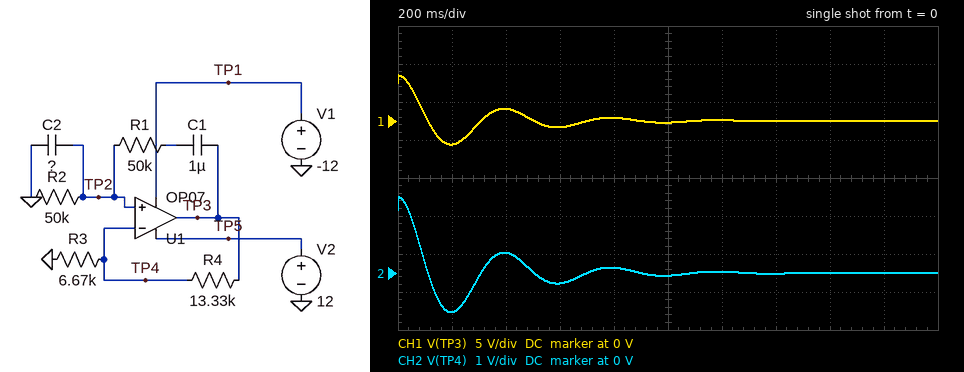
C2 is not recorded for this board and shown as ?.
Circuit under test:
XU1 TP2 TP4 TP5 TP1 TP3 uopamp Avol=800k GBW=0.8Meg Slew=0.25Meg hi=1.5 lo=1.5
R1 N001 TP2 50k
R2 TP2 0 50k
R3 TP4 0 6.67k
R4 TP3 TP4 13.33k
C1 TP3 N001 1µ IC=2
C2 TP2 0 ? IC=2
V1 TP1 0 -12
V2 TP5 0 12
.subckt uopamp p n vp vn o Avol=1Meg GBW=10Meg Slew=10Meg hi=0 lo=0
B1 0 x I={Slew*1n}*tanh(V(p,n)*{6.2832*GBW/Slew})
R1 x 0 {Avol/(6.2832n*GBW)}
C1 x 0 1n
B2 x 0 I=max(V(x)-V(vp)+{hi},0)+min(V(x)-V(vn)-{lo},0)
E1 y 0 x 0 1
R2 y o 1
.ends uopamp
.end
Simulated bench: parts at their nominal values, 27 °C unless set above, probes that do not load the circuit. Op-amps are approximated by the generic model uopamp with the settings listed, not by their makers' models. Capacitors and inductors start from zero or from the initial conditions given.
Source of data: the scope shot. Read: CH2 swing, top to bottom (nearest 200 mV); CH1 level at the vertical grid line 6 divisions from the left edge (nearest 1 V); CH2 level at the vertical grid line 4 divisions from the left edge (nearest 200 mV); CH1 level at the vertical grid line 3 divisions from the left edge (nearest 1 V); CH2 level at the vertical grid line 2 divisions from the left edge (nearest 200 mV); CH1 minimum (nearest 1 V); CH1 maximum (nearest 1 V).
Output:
3.0 V
0 V
200 mV
-1 V
600 mV
-3 V
6 V
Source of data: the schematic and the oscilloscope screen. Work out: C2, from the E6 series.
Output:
1.5 µF
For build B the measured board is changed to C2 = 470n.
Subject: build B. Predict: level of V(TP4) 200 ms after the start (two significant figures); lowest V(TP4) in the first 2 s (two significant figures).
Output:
3.5 V
-3.5 V
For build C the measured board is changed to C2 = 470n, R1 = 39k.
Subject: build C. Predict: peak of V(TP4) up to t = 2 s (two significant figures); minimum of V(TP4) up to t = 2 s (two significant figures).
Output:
3.5 V
-3.5 V
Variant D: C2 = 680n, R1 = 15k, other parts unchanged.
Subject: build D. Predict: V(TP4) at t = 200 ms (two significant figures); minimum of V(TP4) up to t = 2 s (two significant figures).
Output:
3.5 V
-3.5 V
